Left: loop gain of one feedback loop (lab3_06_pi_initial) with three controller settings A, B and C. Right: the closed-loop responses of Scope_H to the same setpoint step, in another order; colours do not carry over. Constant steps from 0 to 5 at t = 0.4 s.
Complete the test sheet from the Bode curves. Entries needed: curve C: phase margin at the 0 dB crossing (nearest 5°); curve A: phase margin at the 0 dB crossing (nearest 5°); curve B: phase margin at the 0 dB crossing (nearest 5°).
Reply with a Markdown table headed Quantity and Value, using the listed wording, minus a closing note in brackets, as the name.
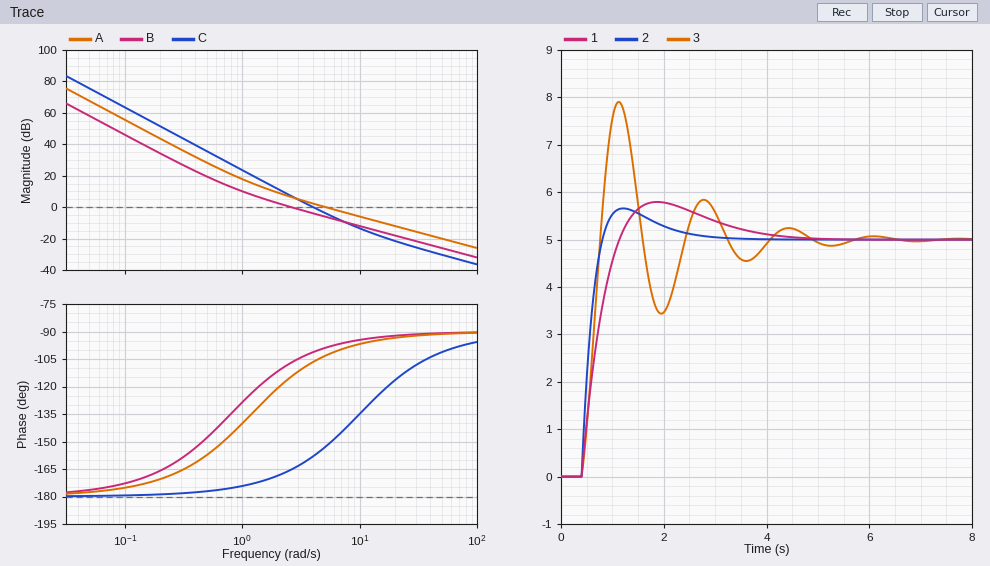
| Quantity | Value |
|---|---|
| curve C: phase margin at the 0 dB crossing | 20° |
| curve A: phase margin at the 0 dB crossing | 75° |
| curve B: phase margin at the 0 dB crossing | 75° |
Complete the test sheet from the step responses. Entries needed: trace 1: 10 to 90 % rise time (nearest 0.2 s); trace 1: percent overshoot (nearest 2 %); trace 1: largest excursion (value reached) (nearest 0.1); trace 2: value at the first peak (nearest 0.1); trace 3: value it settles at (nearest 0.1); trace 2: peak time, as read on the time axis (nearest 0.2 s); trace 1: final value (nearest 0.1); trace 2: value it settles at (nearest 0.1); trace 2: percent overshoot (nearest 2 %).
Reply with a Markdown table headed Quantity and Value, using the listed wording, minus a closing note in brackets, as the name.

| Quantity | Value |
|---|---|
| trace 1: 10 to 90 % rise time | 0.6 s |
| trace 1: percent overshoot | 16 % |
| trace 1: largest excursion (value reached) | 5.8 |
| trace 2: value at the first peak | 5.7 |
| trace 3: value it settles at | 5.0 |
| trace 2: peak time, as read on the time axis | 1.2 s |
| trace 1: final value | 5.0 |
| trace 2: value it settles at | 5.0 |
| trace 2: percent overshoot | 14 % |
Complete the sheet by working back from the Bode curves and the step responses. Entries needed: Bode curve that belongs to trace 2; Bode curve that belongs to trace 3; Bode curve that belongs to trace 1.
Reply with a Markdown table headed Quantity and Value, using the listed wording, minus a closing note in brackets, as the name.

| Quantity | Value |
|---|---|
| Bode curve that belongs to trace 2 | A |
| Bode curve that belongs to trace 3 | C |
| Bode curve that belongs to trace 1 | B |
